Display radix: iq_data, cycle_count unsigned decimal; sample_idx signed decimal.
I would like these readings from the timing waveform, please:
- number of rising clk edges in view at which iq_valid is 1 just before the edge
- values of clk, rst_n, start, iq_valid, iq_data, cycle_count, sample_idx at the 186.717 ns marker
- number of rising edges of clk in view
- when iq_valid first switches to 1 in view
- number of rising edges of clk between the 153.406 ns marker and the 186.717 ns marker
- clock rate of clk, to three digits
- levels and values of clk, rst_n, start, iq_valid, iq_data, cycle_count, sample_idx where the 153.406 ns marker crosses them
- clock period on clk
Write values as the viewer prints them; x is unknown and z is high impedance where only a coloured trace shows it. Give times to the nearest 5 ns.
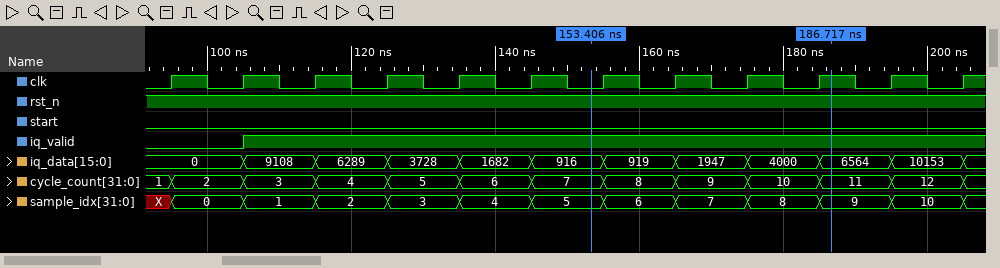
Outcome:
10
clk=1, rst_n=1, start=0, iq_valid=1, iq_data=6564, cycle_count=11, sample_idx=9
12
105 ns
4
100 MHz
clk=0, rst_n=1, start=0, iq_valid=1, iq_data=916, cycle_count=7, sample_idx=5
10 ns
